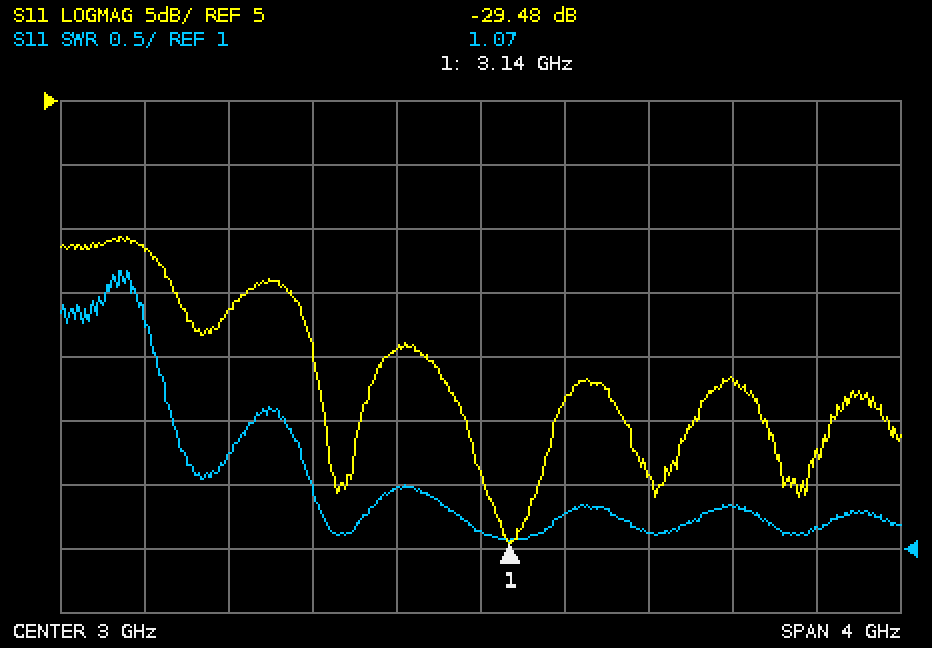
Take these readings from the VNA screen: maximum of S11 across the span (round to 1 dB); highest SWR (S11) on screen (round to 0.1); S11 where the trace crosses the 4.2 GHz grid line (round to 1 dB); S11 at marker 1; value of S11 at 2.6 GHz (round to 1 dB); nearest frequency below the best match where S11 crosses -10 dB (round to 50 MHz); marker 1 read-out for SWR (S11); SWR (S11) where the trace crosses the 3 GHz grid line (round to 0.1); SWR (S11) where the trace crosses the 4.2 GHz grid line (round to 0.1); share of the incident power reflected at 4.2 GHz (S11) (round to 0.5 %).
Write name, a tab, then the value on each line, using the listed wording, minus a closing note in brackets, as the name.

maximum of S11 across the span	-6 dB
highest SWR (S11) on screen	3.2
S11 where the trace crosses the 4.2 GHz grid line	-17 dB
S11 at marker 1	-29.48 dB
value of S11 at 2.6 GHz	-14 dB
nearest frequency below the best match where S11 crosses -10 dB	2.10 GHz
marker 1 read-out for SWR	1.07
SWR (S11) where the trace crosses the 3 GHz grid line	1.1
SWR (S11) where the trace crosses the 4.2 GHz grid line	1.3
share of the incident power reflected at 4.2 GHz (S11)	2.0 %
